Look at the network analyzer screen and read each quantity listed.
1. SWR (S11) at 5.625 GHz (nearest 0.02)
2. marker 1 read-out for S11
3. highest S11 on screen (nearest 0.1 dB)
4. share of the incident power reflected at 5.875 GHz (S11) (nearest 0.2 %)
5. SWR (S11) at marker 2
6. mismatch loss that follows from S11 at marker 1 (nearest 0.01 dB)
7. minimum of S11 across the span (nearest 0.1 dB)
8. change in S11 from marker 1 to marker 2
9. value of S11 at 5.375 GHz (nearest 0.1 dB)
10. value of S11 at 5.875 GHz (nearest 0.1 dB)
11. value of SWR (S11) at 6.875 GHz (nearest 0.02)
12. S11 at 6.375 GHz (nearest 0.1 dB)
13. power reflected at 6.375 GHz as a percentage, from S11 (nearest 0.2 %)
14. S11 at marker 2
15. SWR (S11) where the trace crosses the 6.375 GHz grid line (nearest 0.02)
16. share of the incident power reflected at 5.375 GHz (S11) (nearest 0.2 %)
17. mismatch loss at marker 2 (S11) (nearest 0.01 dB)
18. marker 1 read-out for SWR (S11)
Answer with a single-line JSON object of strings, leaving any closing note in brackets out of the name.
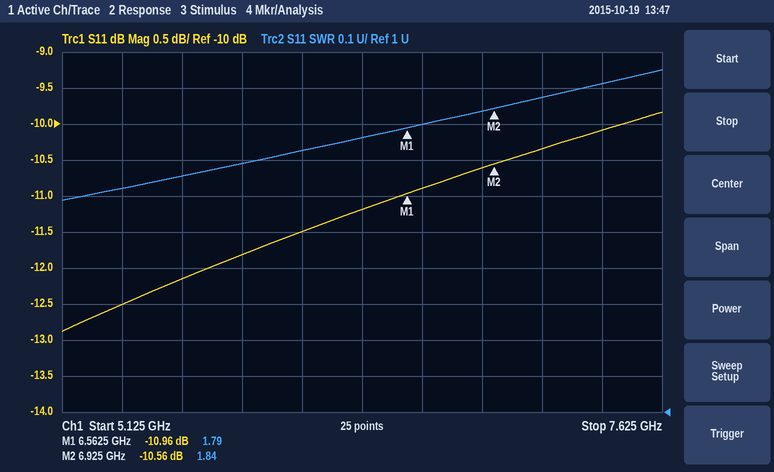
{"SWR (S11) at 5.625 GHz": "1.66", "marker 1 read-out for S11": "-10.96 dB", "highest S11 on screen": "-9.8 dB", "share of the incident power reflected at 5.875 GHz (S11)": "6.6 %", "SWR (S11) at marker 2": "1.84", "mismatch loss that follows from S11 at marker 1": "0.36 dB", "minimum of S11 across the span": "-12.9 dB", "change in S11 from marker 1 to marker 2": "0.40 dB", "value of S11 at 5.375 GHz": "-12.5 dB", "value of S11 at 5.875 GHz": "-11.8 dB", "value of SWR (S11) at 6.875 GHz": "1.84", "S11 at 6.375 GHz": "-11.2 dB", "power reflected at 6.375 GHz as a percentage, from S11": "7.6 %", "S11 at marker 2": "-10.56 dB", "SWR (S11) where the trace crosses the 6.375 GHz grid line": "1.76", "share of the incident power reflected at 5.375 GHz (S11)": "5.6 %", "mismatch loss at marker 2 (S11)": "0.40 dB", "marker 1 read-out for SWR": "1.79"}
